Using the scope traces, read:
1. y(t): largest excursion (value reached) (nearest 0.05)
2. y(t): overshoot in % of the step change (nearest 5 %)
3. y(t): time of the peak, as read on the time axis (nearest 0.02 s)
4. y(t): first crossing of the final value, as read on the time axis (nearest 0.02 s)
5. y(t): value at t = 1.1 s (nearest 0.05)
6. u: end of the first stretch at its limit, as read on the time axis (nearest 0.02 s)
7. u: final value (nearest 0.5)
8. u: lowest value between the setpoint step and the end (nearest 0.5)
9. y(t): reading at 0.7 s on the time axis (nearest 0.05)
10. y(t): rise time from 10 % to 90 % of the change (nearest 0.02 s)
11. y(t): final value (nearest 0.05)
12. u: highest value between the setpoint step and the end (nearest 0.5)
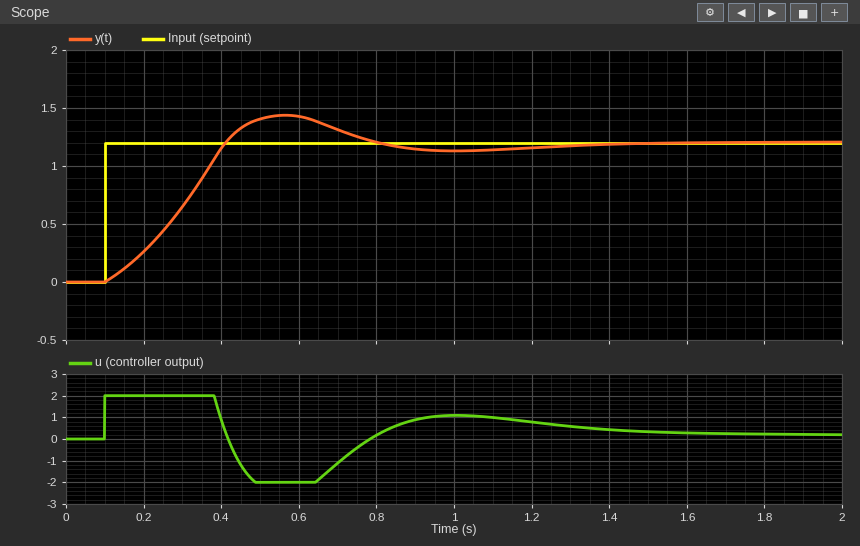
1.45
20 %
0.56 s
0.42 s
1.15
0.38 s
0.0
-2.0
1.30
0.24 s
1.20
2.0
